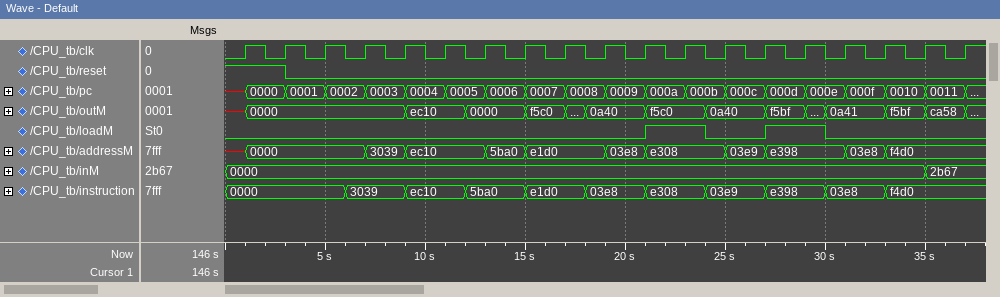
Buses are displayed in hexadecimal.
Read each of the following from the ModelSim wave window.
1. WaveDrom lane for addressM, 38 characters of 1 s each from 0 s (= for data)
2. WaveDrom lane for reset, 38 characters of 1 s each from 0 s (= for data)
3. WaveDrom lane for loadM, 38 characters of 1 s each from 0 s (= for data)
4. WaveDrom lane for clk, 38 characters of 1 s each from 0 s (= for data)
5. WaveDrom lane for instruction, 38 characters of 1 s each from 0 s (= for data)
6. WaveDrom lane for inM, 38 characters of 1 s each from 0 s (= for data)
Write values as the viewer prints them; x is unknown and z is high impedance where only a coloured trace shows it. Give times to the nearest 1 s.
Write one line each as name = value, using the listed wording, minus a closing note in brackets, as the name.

WaveDrom lane for addressM, 38 characters of 1 s each from 0 s = {name: 'addressM', wave: 'x=.....=.=...=.=...=.=...=.=...=.=....', data: '0000 3039 ec10 5ba0 e1d0 03e8 e308 03e9 e398 03e8 f4d0'}
WaveDrom lane for reset, 38 characters of 1 s each from 0 s = {name: 'reset', wave: '1..0..................................'}
WaveDrom lane for loadM, 38 characters of 1 s each from 0 s = {name: 'loadM', wave: '0....................1..0..1..0.......'}
WaveDrom lane for clk, 38 characters of 1 s each from 0 s = {name: 'clk', wave: '01010101010101010101010101010101010101'}
WaveDrom lane for instruction, 38 characters of 1 s each from 0 s = {name: 'instruction', wave: '=.....=..=..=..=..=..=..=..=..=..=....', data: '0000 3039 ec10 5ba0 e1d0 03e8 e308 03e9 e398 03e8 f4d0'}
WaveDrom lane for inM, 38 characters of 1 s each from 0 s = {name: 'inM', wave: '=..................................=..', data: '0000 2b67'}
